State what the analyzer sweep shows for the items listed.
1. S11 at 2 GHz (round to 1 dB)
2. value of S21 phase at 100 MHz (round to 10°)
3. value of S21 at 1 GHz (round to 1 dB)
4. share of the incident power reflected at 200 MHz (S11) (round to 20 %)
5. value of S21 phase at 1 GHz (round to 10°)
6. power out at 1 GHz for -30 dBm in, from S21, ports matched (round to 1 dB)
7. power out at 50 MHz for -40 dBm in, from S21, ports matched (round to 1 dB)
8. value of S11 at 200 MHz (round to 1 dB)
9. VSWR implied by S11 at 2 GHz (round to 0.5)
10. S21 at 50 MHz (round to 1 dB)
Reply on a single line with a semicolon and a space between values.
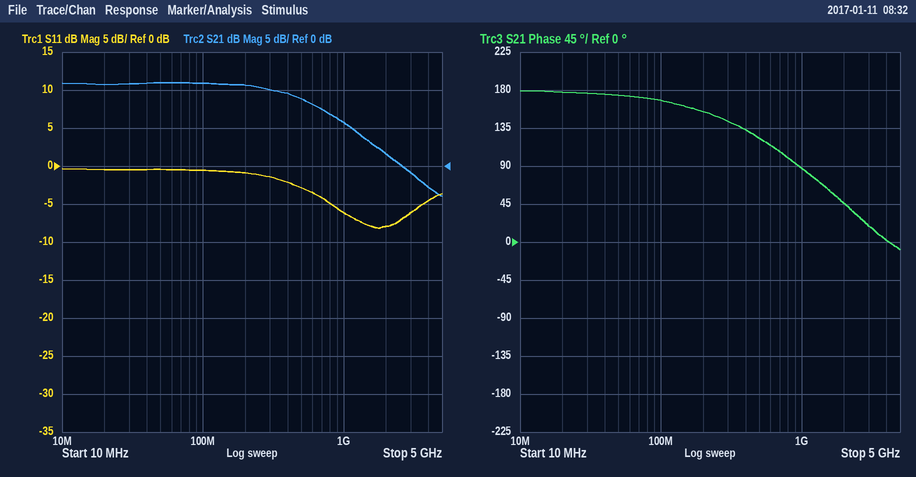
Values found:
-8 dB; 170°; 6 dB; 80 %; 90°; -24 dBm; -29 dBm; -1 dB; 2.5; 11 dB
